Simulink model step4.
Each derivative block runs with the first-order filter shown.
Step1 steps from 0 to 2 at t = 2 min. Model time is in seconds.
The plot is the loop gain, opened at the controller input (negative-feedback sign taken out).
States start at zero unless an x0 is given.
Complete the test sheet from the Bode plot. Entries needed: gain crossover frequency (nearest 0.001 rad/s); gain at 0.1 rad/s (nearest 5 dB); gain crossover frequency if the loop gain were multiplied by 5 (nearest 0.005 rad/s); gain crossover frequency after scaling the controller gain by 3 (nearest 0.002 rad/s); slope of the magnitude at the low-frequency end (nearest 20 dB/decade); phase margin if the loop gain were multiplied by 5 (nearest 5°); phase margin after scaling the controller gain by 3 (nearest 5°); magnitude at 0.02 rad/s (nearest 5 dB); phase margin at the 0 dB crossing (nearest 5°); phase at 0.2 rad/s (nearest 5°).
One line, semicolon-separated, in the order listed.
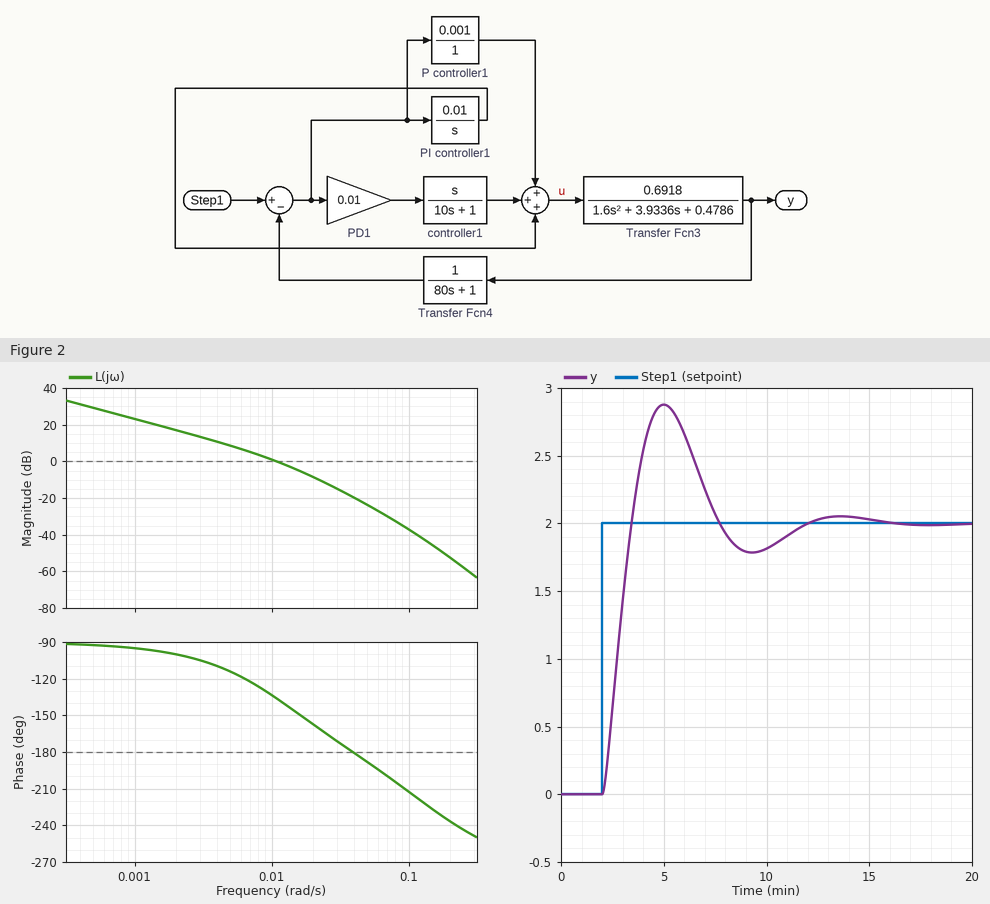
0.011 rad/s; -35 dB; 0.030 rad/s; 0.022 rad/s; -20 dB/decade; 10°; 20°; -10 dB; 45°; -235°
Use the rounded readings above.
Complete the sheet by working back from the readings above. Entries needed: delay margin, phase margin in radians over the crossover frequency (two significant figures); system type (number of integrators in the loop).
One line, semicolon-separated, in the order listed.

71 s; 1
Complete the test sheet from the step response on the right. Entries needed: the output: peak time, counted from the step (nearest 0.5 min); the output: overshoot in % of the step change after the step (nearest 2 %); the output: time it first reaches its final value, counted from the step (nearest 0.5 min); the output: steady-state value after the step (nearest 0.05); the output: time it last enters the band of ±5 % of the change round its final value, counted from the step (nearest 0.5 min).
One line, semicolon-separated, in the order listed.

3.0 min; 44 %; 1.5 min; 2.00; 9.0 min
